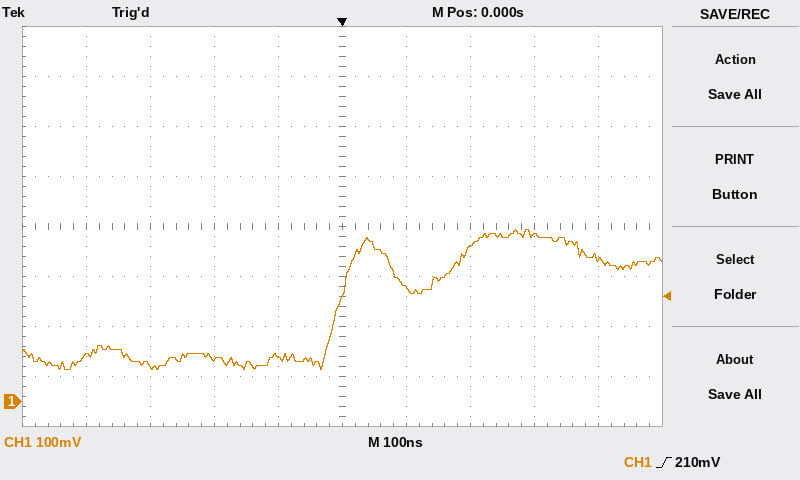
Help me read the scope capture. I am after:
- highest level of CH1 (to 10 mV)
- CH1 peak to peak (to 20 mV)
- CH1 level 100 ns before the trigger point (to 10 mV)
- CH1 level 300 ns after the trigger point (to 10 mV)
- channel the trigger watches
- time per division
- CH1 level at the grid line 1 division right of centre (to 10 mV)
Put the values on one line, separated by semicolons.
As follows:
340 mV; 280 mV; 90 mV; 330 mV; CH1; 100 ns; 230 mV
